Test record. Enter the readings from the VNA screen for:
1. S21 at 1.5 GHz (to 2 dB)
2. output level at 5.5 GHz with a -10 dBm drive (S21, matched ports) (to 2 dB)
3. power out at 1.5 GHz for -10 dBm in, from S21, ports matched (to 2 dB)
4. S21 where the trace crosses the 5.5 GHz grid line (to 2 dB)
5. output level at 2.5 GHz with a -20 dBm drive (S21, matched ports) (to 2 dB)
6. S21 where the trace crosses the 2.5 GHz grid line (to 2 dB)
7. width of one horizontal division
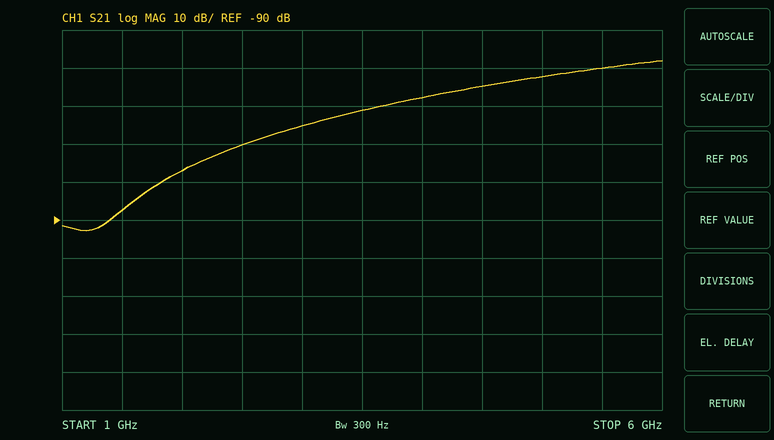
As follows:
-88 dB
-60 dBm
-98 dBm
-50 dB
-90 dBm
-70 dB
500 MHz
